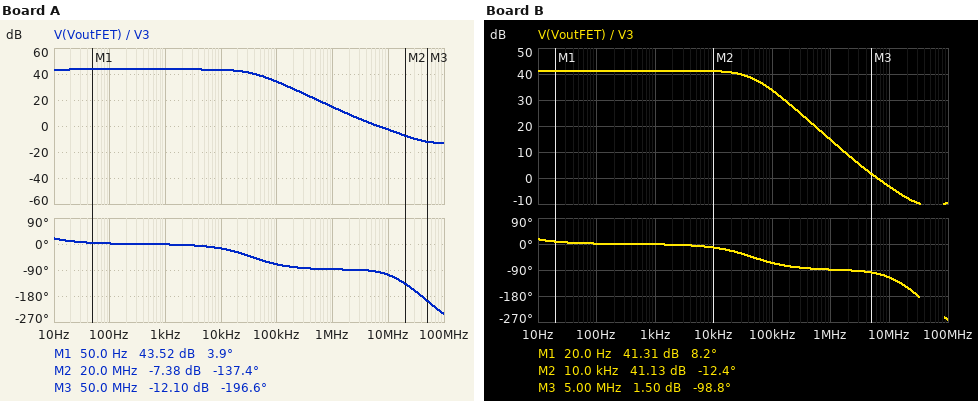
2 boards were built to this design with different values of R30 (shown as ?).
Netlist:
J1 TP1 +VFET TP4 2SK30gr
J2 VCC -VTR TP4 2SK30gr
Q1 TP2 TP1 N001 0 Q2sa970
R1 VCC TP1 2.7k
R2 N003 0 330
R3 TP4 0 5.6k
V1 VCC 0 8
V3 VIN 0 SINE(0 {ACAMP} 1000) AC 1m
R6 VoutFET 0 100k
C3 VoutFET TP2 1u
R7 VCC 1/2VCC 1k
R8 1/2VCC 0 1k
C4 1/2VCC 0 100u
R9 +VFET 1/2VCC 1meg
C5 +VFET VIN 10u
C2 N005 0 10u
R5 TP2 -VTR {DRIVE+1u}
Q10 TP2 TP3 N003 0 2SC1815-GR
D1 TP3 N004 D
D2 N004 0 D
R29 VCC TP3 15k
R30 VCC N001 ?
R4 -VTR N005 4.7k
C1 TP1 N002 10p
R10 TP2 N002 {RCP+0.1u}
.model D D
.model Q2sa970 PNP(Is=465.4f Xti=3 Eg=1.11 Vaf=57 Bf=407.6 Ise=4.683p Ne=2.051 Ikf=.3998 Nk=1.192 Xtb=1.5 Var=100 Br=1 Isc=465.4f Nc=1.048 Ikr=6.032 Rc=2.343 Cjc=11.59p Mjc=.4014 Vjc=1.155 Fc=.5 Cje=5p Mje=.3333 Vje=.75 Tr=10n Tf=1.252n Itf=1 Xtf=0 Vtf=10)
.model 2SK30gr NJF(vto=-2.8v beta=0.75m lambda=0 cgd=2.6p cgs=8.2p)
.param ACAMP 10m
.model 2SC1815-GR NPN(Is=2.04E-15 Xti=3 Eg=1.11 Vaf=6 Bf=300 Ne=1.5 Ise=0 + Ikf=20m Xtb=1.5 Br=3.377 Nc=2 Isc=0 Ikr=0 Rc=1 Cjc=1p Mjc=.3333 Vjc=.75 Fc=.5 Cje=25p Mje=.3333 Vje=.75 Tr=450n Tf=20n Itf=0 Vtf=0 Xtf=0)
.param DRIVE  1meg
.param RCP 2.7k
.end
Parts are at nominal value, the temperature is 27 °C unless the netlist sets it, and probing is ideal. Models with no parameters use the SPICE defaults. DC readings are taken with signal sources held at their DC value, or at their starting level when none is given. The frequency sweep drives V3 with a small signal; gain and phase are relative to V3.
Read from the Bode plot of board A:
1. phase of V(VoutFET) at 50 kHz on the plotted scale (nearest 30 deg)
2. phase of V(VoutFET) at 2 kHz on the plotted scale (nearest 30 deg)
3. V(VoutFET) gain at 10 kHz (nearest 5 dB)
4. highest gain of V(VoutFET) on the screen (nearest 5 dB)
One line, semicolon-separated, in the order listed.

-60 deg; 0 deg; 45 dB; 45 dB
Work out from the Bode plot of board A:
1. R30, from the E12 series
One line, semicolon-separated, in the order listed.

150 Ω
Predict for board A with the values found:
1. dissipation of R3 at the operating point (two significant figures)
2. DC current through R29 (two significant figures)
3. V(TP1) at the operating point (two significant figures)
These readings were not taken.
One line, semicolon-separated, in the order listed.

6.8 mW; 450 µA; 7.2 V
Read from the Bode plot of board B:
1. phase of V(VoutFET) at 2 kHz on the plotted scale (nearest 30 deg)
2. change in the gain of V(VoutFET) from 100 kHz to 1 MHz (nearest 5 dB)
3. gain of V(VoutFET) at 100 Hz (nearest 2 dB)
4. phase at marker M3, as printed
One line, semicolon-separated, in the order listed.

0 deg; -20 dB; 42 dB; -98.8 deg
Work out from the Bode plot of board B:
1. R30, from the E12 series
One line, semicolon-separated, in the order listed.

330 Ω
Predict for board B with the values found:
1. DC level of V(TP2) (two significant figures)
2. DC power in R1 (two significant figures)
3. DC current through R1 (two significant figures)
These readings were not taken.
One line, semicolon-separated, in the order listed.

4.2 V; 480 µW; 420 µA
